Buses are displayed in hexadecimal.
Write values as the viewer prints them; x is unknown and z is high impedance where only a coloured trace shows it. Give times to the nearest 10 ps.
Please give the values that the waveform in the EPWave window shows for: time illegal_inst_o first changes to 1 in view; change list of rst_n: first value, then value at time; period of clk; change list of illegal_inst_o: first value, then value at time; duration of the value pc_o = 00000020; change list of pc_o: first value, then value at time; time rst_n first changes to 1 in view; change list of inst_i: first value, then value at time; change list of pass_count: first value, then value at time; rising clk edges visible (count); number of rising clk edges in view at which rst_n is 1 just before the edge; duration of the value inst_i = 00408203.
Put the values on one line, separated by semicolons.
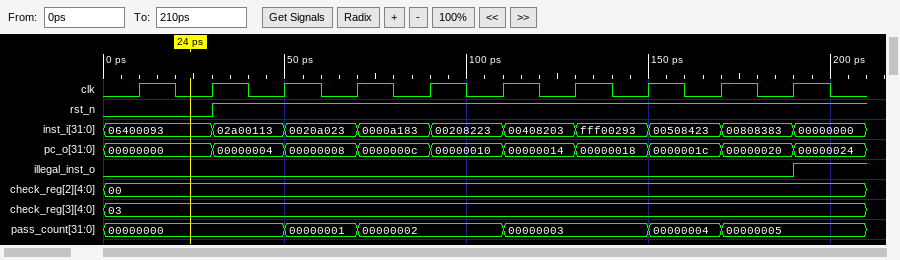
190 ps; 0, 1 at 30 ps; 20 ps; 0, 1 at 190 ps; 20 ps; 00000000, 00000004 at 30 ps, 00000008 at 50 ps, 0000000c at 70 ps, 00000010 at 90 ps, 00000014 at 110 ps, 00000018 at 130 ps, 0000001c at 150 ps, 00000020 at 170 ps, 00000024 at 190 ps; 30 ps; 06400093, 02a00113 at 30 ps, 0020a023 at 50 ps, 0000a183 at 70 ps, 00208223 at 90 ps, 00408203 at 110 ps, fff00293 at 130 ps, 00508423 at 150 ps, 00808383 at 170 ps, 00000000 at 190 ps; 00000000, 00000001 at 50 ps, 00000002 at 70 ps, 00000003 at 110 ps, 00000004 at 150 ps, 00000005 at 170 ps; 10; 8; 20 ps
